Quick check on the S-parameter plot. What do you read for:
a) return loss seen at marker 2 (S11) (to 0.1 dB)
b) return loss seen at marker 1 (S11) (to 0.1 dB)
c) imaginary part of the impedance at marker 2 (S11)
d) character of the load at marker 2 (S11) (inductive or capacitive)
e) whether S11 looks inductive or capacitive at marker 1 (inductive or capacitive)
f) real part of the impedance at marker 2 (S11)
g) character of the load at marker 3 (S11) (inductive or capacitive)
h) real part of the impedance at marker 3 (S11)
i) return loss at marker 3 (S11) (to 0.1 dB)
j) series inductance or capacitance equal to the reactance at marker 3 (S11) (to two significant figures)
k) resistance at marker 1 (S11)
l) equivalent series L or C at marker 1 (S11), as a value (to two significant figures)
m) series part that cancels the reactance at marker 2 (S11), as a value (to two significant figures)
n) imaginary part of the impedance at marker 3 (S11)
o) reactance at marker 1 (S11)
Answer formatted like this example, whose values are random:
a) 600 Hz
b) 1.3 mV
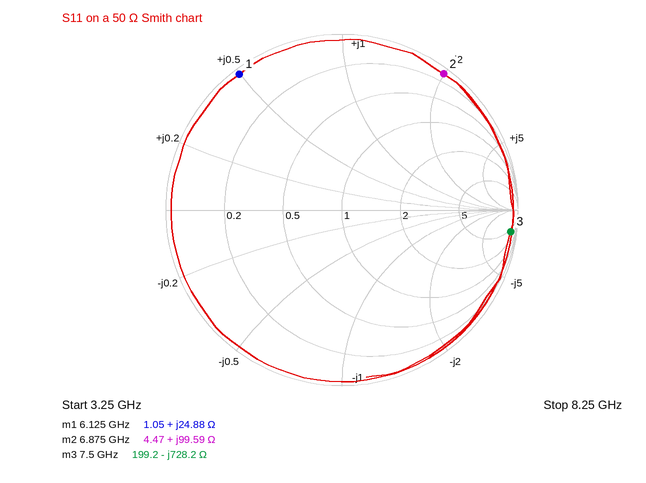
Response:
a) 0.3 dB
b) 0.3 dB
c) +99.59 Ω
d) inductive
e) inductive
f) 4.47 Ω
g) capacitive
h) 199.2 Ω
i) 0.3 dB
j) 29 fF
k) 1.05 Ω
l) 650 pH
m) 230 fF
n) -728.2 Ω
o) +24.88 Ω
